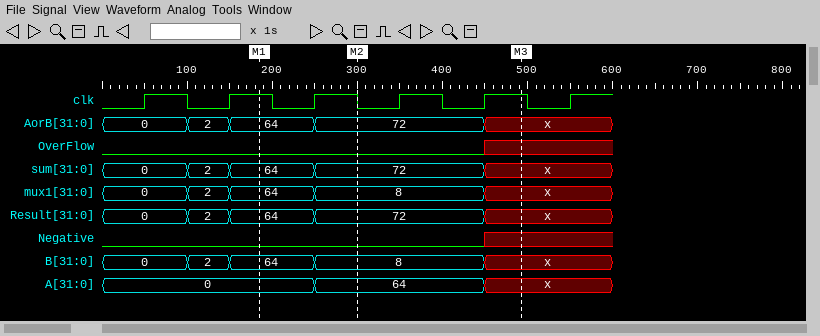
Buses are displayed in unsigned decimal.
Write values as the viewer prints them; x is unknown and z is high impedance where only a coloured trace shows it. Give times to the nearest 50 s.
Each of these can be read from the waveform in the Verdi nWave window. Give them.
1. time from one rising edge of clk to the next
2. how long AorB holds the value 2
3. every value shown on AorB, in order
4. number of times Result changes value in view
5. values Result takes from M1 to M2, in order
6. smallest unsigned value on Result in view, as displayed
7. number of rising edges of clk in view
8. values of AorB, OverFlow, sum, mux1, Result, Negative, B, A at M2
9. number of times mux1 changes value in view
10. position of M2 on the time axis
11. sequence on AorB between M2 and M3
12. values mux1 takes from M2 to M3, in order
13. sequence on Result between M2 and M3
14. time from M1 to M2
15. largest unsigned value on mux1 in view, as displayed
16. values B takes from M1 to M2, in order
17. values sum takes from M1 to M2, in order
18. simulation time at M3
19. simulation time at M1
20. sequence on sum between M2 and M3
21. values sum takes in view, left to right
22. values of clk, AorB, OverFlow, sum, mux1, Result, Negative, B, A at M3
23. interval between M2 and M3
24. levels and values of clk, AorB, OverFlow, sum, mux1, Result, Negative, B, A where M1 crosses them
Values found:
100 s
50 s
0, 2, 64, 72, x
4
64, 72
0
6
AorB=72, OverFlow=0, sum=72, mux1=8, Result=72, Negative=0, B=8, A=64
4
300 s
72, x
8, x
72, x
100 s
64
64, 8
64, 72
500 s
200 s
72, x
0, 2, 64, 72, x
clk=1, AorB=x, OverFlow=x, sum=x, mux1=x, Result=x, Negative=x, B=x, A=x
200 s
clk=1, AorB=64, OverFlow=0, sum=64, mux1=64, Result=64, Negative=0, B=64, A=0
